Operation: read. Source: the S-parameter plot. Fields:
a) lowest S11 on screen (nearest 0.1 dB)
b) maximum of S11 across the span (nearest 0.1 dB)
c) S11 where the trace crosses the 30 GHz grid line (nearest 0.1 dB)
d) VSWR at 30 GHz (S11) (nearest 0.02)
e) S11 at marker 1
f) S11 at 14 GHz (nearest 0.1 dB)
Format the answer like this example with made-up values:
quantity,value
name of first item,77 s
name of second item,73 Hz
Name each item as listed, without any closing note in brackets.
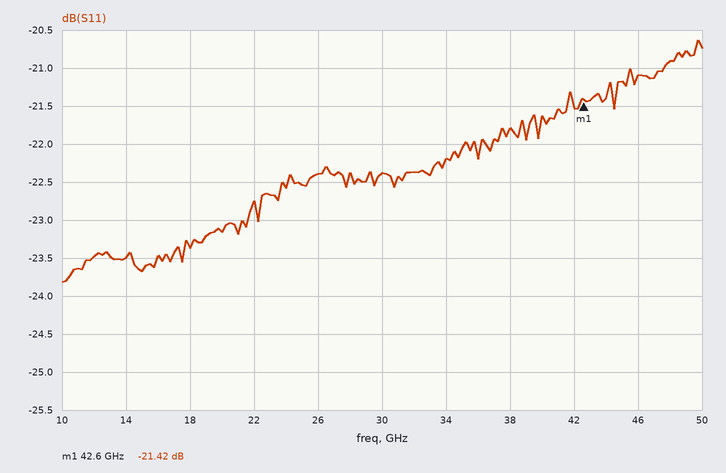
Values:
quantity,value
lowest S11 on screen,-23.8 dB
maximum of S11 across the span,-20.6 dB
S11 where the trace crosses the 30 GHz grid line,-22.4 dB
VSWR at 30 GHz (S11),1.16
S11 at marker 1,-21.42 dB
S11 at 14 GHz,-23.5 dB
